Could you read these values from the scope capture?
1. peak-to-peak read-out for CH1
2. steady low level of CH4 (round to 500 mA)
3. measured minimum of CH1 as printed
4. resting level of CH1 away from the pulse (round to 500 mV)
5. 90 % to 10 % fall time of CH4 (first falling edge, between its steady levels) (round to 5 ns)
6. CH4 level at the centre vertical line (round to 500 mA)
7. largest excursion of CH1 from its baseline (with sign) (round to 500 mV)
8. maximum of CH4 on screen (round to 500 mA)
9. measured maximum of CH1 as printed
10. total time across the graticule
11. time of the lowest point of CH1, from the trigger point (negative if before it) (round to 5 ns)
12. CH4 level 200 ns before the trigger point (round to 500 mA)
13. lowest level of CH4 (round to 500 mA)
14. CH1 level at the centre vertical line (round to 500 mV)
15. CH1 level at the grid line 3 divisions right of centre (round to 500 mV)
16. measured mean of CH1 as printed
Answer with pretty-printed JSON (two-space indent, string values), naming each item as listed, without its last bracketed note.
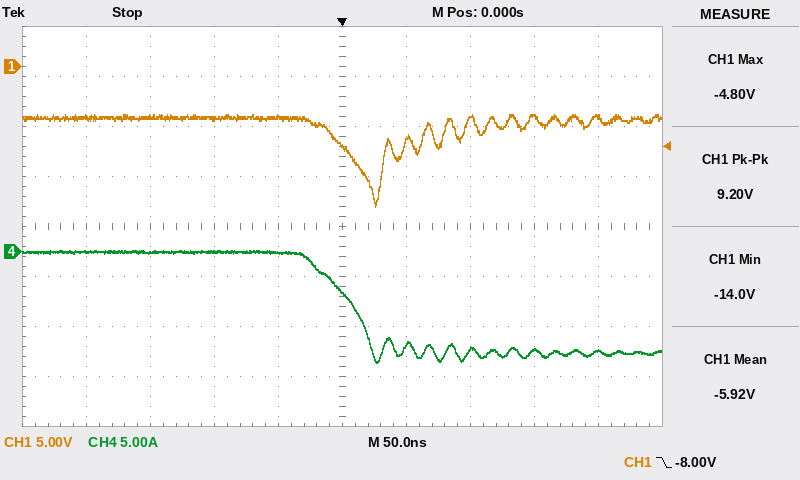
{
  "peak-to-peak read-out for CH1": "9.20 V",
  "steady low level of CH4": "-10.0 A",
  "measured minimum of CH1 as printed": "-14.0 V",
  "resting level of CH1 away from the pulse": "-5.0 V",
  "90 % to 10 % fall time of CH4 (first falling edge, between its steady levels)": "45 ns",
  "CH4 level at the centre vertical line": "-4.0 A",
  "largest excursion of CH1 from its baseline (with sign)": "-9.0 V",
  "maximum of CH4 on screen": "0.0 A",
  "measured maximum of CH1 as printed": "-4.80 V",
  "total time across the graticule": "500 ns",
  "time of the lowest point of CH1, from the trigger point (negative if before it)": "+25 ns",
  "CH4 level 200 ns before the trigger point": "0.0 A",
  "lowest level of CH4": "-11.0 A",
  "CH1 level at the centre vertical line": "-8.0 V",
  "CH1 level at the grid line 3 divisions right of centre": "-5.0 V",
  "measured mean of CH1 as printed": "-5.92 V"
}
